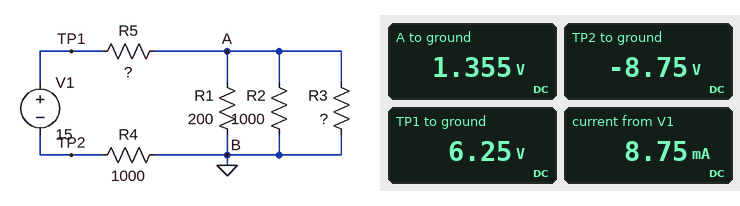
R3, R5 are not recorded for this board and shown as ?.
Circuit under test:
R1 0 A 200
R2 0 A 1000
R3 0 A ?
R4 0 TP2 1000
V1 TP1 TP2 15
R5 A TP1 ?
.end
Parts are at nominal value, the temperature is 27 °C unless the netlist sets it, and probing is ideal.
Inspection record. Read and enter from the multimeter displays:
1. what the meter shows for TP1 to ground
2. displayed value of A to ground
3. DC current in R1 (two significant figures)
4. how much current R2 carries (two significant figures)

6.25 V
1.355 V
6.8 mA
1.4 mA
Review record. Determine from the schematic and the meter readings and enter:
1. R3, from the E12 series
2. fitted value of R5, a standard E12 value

2.2 kΩ
560 Ω
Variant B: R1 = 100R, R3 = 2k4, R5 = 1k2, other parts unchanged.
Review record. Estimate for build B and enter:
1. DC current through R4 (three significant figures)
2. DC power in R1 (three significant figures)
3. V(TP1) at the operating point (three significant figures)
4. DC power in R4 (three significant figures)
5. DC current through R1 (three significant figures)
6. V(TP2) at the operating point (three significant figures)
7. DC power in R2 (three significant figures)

6.56 mA
3.30 mW
8.44 V
43.0 mW
5.74 mA
-6.56 V
330 µW
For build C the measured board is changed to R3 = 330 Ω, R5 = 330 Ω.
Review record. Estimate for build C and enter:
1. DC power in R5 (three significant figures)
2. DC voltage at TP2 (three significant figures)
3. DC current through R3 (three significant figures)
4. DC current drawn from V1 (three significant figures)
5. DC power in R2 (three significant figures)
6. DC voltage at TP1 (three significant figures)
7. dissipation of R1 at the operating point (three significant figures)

35.8 mW
-10.4 V
3.49 mA
10.4 mA
1.33 mW
4.59 V
6.65 mW
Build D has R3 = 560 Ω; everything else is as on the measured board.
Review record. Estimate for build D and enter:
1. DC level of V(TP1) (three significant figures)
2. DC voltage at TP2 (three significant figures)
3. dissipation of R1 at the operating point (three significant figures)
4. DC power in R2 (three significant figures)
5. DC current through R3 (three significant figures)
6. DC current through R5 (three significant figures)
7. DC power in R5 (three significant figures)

6.12 V
-8.88 V
6.51 mW
1.30 mW
2.04 mA
8.88 mA
44.2 mW
